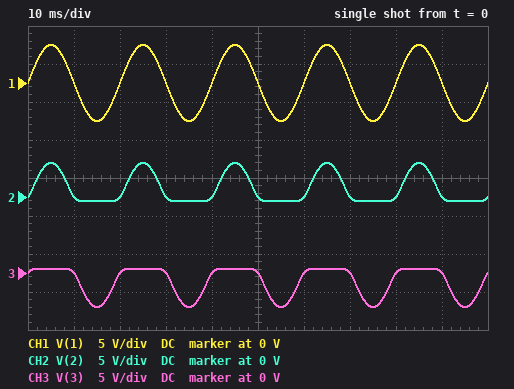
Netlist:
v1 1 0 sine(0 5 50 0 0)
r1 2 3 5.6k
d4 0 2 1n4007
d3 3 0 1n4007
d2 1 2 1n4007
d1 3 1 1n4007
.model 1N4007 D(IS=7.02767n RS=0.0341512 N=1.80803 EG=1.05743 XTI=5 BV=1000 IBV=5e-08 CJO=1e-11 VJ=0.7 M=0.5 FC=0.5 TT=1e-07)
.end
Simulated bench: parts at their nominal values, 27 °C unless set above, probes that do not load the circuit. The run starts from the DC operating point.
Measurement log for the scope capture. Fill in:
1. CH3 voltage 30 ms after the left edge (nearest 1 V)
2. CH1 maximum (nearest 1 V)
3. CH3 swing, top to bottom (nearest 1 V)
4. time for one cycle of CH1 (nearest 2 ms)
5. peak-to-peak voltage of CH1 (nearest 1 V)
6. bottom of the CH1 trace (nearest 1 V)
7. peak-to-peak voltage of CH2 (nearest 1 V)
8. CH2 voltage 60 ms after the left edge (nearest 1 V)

0 V
5 V
5 V
20 ms
10 V
-5 V
5 V
0 V
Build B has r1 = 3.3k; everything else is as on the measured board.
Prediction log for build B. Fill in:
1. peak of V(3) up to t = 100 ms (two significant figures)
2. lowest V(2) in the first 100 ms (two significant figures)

560 mV
-560 mV
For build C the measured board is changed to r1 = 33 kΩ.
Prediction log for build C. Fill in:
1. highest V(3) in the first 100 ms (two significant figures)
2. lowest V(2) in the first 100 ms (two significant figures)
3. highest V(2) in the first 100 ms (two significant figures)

460 mV
-460 mV
4.5 V
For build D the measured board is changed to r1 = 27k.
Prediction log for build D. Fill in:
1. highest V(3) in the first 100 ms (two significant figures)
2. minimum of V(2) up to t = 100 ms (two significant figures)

470 mV
-470 mV
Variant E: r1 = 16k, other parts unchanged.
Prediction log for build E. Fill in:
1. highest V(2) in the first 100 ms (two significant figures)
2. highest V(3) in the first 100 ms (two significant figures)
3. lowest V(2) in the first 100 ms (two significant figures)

4.5 V
490 mV
-490 mV
